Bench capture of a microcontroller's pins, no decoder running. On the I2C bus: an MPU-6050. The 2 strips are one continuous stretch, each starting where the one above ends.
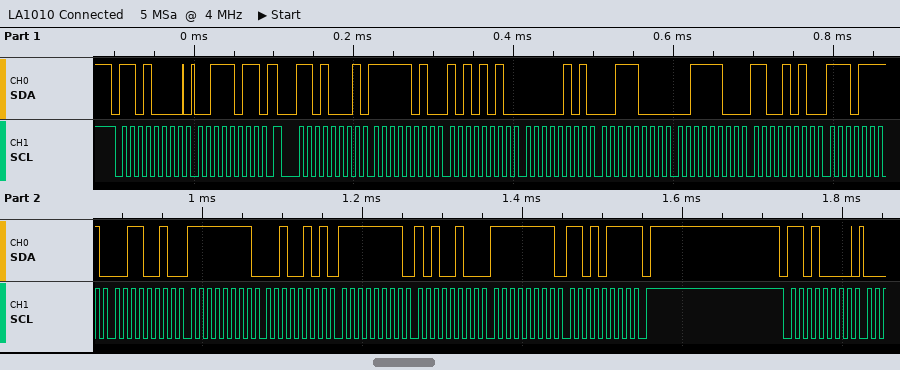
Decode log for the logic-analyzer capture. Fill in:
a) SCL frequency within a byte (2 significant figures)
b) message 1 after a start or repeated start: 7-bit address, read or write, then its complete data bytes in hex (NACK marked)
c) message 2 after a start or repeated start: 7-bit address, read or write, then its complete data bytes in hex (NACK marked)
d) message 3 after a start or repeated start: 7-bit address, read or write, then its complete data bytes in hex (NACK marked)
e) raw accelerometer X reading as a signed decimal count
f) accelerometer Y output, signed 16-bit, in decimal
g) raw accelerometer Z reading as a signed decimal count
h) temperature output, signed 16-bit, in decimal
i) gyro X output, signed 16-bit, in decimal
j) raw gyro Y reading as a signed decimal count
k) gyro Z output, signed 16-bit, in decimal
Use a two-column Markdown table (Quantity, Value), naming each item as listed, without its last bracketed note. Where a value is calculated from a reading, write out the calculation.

| Quantity | Value |
|---|---|
| SCL frequency within a byte | 100 kHz |
| message 1 after a start or repeated start: 7-bit address, read or write, then its complete data bytes in hex | 0x68 write: 3B |
| message 2 after a start or repeated start: 7-bit address, read or write, then its complete data bytes in hex | 0x68 read: FA AA 05 38 3C CA EF 32 FF 25 FF A4 FF D7 NACK |
| message 3 after a start or repeated start: 7-bit address, read or write, then its complete data bytes in hex | 0x68 write |
| raw accelerometer X reading as a signed decimal count | 0xFAAA = -1366 |
| accelerometer Y output, signed 16-bit, in decimal | 0x0538 = 1336 |
| raw accelerometer Z reading as a signed decimal count | 0x3CCA = 15562 |
| temperature output, signed 16-bit, in decimal | 0xEF32 = -4302 |
| gyro X output, signed 16-bit, in decimal | 0xFF25 = -219 |
| raw gyro Y reading as a signed decimal count | 0xFFA4 = -92 |
| gyro Z output, signed 16-bit, in decimal | 0xFFD7 = -41 |
